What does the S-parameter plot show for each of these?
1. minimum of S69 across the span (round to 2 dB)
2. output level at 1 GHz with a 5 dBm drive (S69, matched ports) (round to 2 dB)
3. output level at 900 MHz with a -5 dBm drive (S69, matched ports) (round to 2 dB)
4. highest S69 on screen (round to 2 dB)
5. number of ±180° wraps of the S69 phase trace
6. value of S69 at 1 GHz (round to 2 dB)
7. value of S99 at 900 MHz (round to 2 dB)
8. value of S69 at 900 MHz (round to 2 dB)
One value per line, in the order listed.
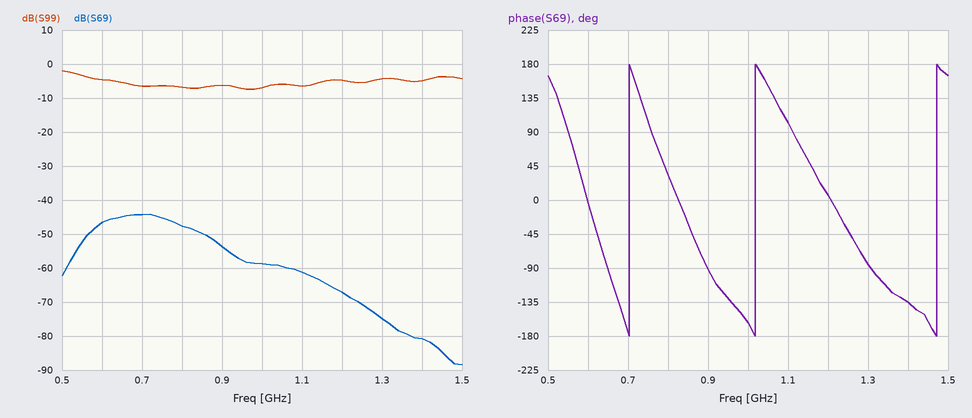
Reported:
-88 dB
-54 dBm
-58 dBm
-44 dB
3
-58 dB
-6 dB
-54 dB
